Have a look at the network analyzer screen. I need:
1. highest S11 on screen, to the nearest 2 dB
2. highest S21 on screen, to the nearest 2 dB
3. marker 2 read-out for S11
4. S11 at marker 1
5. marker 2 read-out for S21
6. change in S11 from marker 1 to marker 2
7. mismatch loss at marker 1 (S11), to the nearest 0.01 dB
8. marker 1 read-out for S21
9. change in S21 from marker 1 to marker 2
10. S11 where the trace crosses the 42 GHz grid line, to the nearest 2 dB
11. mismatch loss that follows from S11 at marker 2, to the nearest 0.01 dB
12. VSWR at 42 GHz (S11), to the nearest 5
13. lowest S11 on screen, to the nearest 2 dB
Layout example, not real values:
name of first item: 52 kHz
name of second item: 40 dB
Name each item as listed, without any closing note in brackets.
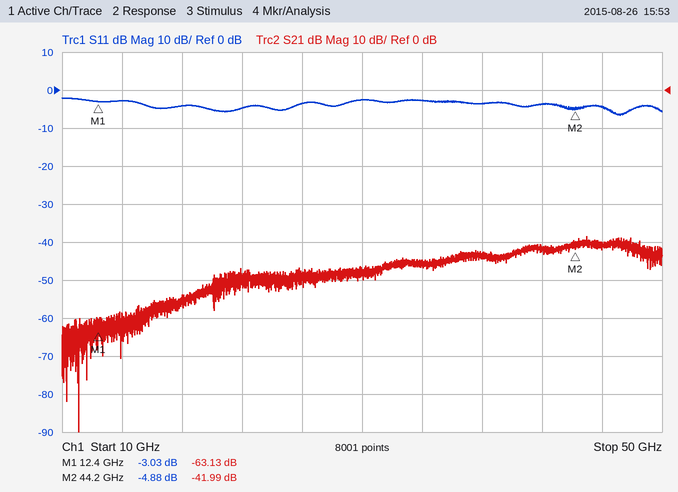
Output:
highest S11 on screen, to the nearest 2 dB: -2 dB
highest S21 on screen, to the nearest 2 dB: -38 dB
marker 2 read-out for S11: -4.88 dB
S11 at marker 1: -3.03 dB
marker 2 read-out for S21: -41.99 dB
change in S11 from marker 1 to marker 2: -1.85 dB
mismatch loss at marker 1 (S11), to the nearest 0.01 dB: 2.99 dB
marker 1 read-out for S21: -63.13 dB
change in S21 from marker 1 to marker 2: 21.14 dB
S11 where the trace crosses the 42 GHz grid line, to the nearest 2 dB: -4 dB
mismatch loss that follows from S11 at marker 2, to the nearest 0.01 dB: 1.71 dB
VSWR at 42 GHz (S11), to the nearest 5: 5
lowest S11 on screen, to the nearest 2 dB: -6 dB
